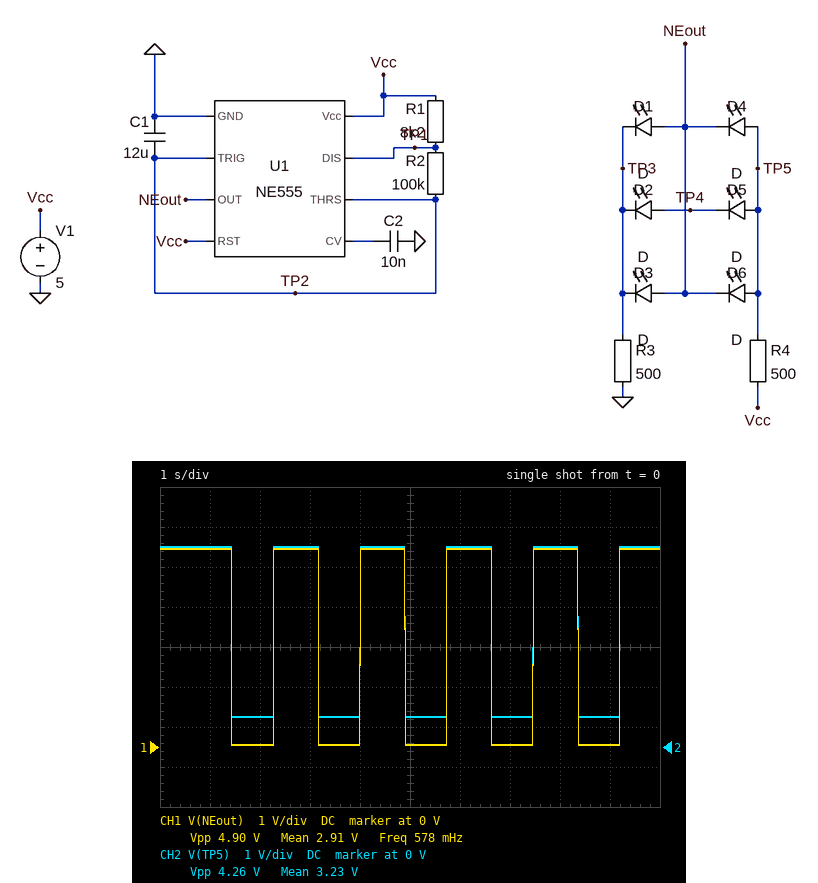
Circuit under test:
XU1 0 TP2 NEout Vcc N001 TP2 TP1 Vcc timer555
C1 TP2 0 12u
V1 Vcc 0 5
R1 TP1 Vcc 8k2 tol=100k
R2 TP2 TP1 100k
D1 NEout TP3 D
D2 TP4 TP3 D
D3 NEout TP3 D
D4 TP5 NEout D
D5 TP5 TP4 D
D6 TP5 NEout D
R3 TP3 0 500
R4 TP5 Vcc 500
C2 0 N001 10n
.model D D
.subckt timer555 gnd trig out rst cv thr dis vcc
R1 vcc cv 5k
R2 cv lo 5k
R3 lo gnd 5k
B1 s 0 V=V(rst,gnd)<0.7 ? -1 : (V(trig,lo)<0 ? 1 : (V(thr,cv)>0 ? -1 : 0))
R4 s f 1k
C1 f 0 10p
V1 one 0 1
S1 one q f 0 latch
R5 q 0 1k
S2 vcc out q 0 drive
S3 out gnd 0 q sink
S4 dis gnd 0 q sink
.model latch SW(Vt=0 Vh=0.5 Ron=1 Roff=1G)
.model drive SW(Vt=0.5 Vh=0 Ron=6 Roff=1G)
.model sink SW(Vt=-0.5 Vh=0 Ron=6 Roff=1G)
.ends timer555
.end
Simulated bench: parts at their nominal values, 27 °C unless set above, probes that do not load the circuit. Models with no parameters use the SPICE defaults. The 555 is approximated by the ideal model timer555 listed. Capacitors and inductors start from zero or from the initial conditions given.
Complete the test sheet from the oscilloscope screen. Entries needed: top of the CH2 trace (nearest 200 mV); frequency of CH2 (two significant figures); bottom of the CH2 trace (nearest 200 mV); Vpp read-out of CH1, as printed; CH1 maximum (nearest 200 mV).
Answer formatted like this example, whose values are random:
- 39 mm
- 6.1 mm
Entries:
- 5.0 V
- 580 mHz
- 800 mV
- 4.90 V
- 5.0 V
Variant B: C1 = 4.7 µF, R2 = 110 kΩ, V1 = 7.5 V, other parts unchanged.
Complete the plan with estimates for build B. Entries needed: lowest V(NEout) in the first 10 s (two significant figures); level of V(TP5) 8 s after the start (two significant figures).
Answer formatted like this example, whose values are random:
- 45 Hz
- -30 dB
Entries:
- 81 mV
- 7.5 V
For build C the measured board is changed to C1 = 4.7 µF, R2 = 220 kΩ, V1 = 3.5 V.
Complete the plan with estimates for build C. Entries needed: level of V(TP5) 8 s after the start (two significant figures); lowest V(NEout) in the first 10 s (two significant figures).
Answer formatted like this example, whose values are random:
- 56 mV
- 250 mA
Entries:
- 3.5 V
- 33 mV
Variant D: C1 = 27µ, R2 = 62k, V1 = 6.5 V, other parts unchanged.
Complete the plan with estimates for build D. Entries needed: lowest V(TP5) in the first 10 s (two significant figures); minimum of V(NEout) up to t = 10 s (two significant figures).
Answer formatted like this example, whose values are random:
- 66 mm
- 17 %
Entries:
- 770 mV
- 69 mV
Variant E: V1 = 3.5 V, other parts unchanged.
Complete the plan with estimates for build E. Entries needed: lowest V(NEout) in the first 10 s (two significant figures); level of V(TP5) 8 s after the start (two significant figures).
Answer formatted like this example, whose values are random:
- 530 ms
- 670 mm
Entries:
- 33 mV
- 3.5 V
